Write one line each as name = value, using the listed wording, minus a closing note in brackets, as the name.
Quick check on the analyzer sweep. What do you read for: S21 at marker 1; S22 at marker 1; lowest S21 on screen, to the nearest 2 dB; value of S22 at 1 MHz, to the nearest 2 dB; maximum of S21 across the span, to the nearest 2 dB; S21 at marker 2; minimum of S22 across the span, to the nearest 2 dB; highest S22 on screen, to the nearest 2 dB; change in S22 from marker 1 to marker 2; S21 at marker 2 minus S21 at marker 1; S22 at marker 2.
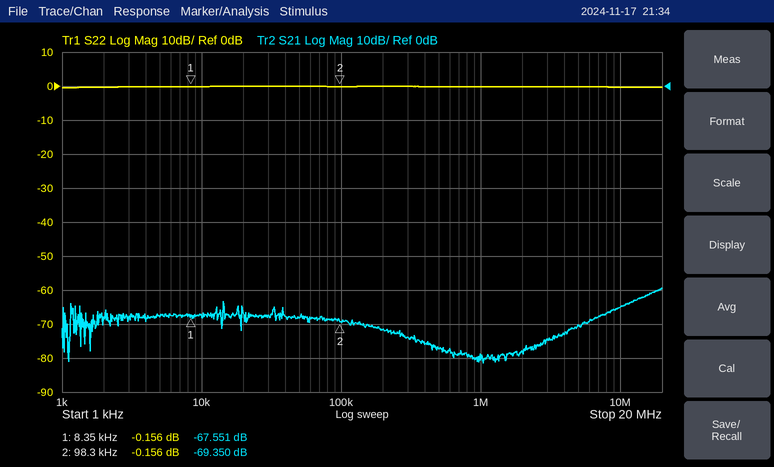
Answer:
S21 at marker 1 = -67.551 dB
S22 at marker 1 = -0.156 dB
lowest S21 on screen, to the nearest 2 dB = -82 dB
value of S22 at 1 MHz, to the nearest 2 dB = 0 dB
maximum of S21 across the span, to the nearest 2 dB = -60 dB
S21 at marker 2 = -69.350 dB
minimum of S22 across the span, to the nearest 2 dB = 0 dB
highest S22 on screen, to the nearest 2 dB = 0 dB
change in S22 from marker 1 to marker 2 = 0.000 dB
S21 at marker 2 minus S21 at marker 1 = -1.799 dB
S22 at marker 2 = -0.156 dB
